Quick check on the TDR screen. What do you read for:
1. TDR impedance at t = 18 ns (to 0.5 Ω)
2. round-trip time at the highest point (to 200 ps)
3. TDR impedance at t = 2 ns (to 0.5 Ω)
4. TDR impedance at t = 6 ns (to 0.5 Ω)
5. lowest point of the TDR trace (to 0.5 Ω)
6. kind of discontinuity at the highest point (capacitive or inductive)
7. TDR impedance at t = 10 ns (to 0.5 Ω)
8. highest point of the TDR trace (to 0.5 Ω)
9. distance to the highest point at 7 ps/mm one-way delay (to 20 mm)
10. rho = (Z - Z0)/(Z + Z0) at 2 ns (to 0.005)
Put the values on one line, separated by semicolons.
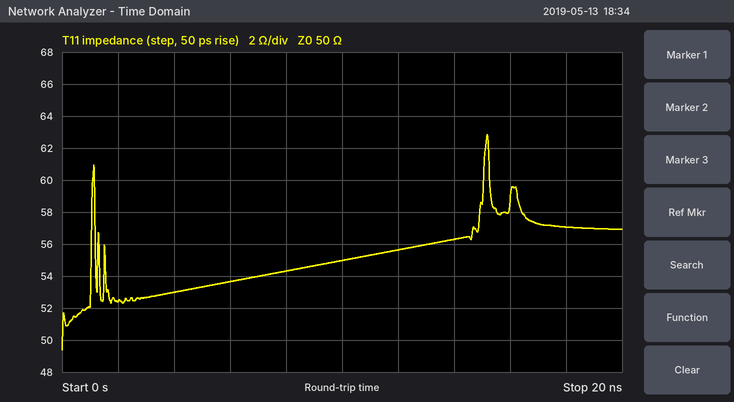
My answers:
57.0 Ω; 15.2 ns; 52.5 Ω; 53.5 Ω; 49.5 Ω; inductive; 55.0 Ω; 63.0 Ω; 1.08 m; +0.025
